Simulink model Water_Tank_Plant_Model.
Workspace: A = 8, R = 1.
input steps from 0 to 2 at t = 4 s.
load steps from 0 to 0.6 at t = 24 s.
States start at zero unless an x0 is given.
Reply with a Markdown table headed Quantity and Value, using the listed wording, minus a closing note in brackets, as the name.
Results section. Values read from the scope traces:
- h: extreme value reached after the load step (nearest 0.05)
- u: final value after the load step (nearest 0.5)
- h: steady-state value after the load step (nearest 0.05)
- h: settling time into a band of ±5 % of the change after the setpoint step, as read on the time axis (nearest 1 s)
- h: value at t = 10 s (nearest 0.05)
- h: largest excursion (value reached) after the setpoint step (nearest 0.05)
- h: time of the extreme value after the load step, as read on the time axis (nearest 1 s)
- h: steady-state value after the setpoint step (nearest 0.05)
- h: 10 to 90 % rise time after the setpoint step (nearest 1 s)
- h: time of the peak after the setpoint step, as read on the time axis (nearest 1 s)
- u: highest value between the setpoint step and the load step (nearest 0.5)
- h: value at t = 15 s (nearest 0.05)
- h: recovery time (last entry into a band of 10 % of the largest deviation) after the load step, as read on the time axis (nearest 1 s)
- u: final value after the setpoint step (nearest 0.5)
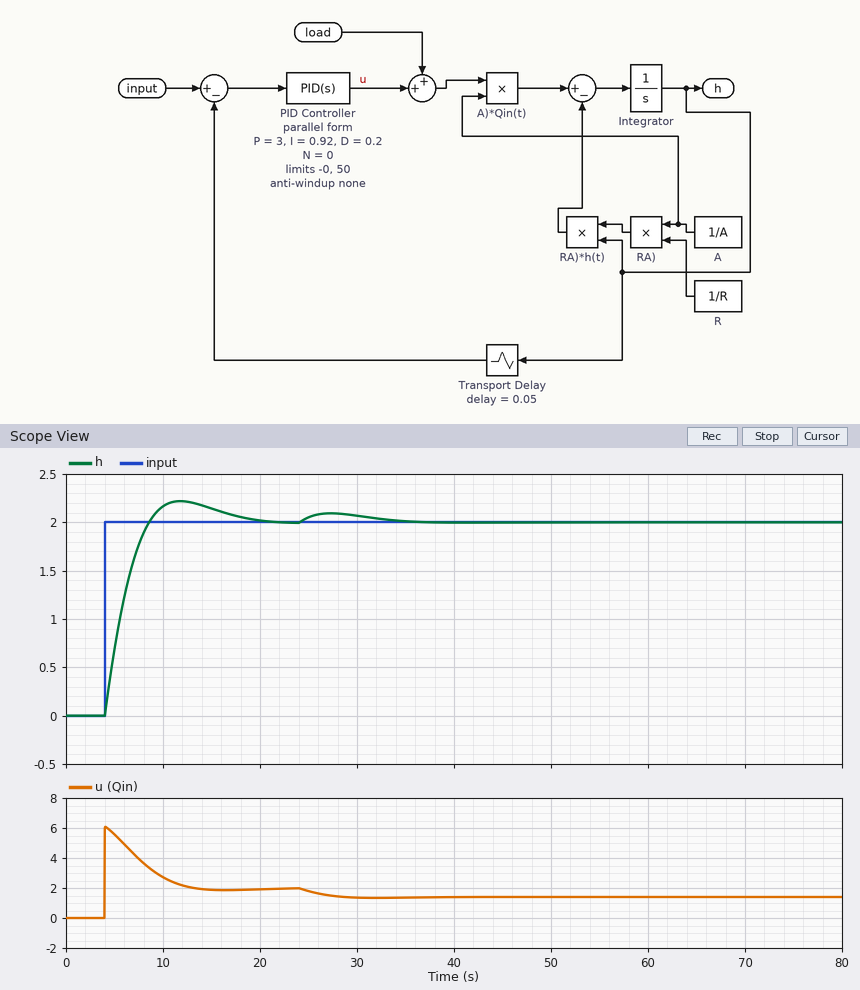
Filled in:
| Quantity | Value |
|---|---|
| h: extreme value reached after the load step | 2.10 |
| u: final value after the load step | 1.5 |
| h: steady-state value after the load step | 2.00 |
| h: settling time into a band of ±5 % of the change after the setpoint step, as read on the time axis | 16 s |
| h: value at t = 10 s | 2.15 |
| h: largest excursion (value reached) after the setpoint step | 2.20 |
| h: time of the extreme value after the load step, as read on the time axis | 27 s |
| h: steady-state value after the setpoint step | 2.00 |
| h: 10 to 90 % rise time after the setpoint step | 3 s |
| h: time of the peak after the setpoint step, as read on the time axis | 12 s |
| u: highest value between the setpoint step and the load step | 6.0 |
| h: value at t = 15 s | 2.15 |
| h: recovery time (last entry into a band of 10 % of the largest deviation) after the load step, as read on the time axis | 35 s |
| u: final value after the setpoint step | 2.0 |
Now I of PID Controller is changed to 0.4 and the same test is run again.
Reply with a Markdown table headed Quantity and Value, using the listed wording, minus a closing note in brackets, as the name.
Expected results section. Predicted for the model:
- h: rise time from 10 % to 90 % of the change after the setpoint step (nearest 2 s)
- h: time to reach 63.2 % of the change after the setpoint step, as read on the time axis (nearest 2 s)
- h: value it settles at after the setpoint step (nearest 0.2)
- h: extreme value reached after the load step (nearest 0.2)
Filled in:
| Quantity | Value |
|---|---|
| h: rise time from 10 % to 90 % of the change after the setpoint step | 6 s |
| h: time to reach 63.2 % of the change after the setpoint step, as read on the time axis | 6 s |
| h: value it settles at after the setpoint step | 2.0 |
| h: extreme value reached after the load step | 2.2 |
